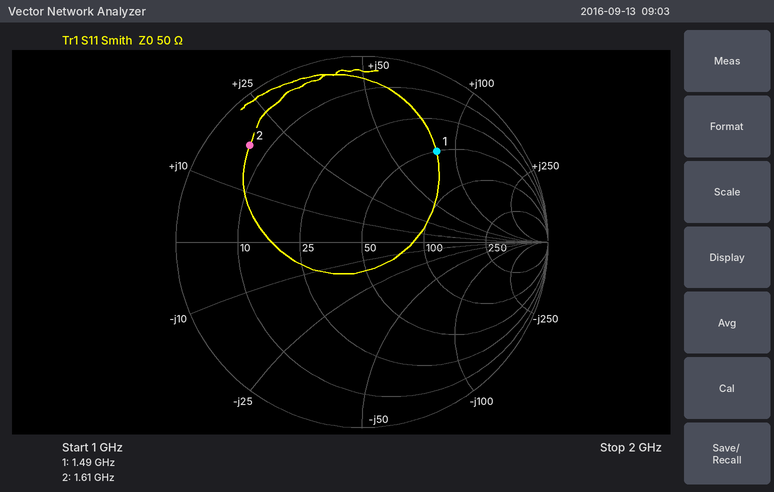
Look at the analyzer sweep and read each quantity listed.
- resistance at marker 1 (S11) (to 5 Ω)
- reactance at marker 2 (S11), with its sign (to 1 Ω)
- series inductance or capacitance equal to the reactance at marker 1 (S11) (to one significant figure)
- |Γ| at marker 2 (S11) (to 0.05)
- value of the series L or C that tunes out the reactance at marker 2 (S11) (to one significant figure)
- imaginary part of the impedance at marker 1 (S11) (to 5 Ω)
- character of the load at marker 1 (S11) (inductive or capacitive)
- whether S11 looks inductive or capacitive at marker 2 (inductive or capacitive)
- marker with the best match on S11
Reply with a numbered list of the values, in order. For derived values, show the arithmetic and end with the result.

1. 50 Ω
2. +18 Ω
3. L = 80 Ω/(2π × 1.49 GHz) ≈ 9 nH
4. 0.80
5. C = 1/(2π × 1.61 GHz × 18 Ω) ≈ 5 pF
6. +80 Ω
7. inductive
8. inductive
9. marker 1
